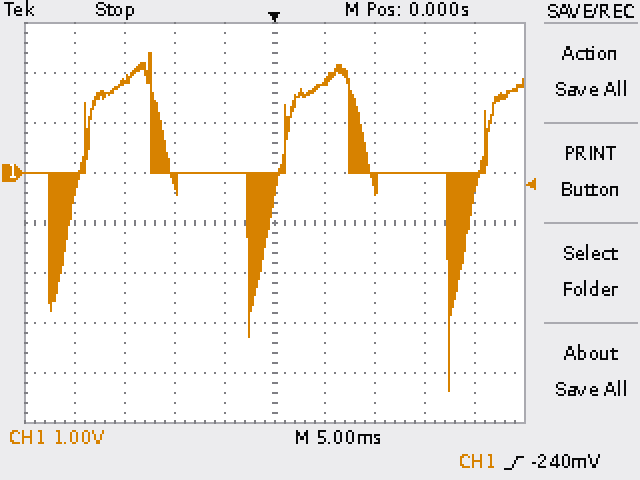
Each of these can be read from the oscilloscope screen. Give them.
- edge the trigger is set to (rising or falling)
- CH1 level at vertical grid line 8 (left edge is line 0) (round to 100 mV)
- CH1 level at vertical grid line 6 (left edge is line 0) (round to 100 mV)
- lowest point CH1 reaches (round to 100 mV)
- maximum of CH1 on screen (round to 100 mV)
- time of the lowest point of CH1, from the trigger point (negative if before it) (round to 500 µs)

rising
0.0 V
1.8 V
-4.4 V
2.4 V
+17.5 ms
